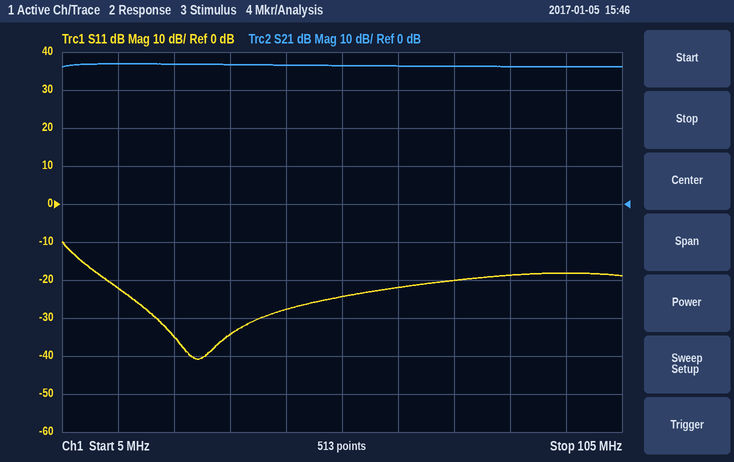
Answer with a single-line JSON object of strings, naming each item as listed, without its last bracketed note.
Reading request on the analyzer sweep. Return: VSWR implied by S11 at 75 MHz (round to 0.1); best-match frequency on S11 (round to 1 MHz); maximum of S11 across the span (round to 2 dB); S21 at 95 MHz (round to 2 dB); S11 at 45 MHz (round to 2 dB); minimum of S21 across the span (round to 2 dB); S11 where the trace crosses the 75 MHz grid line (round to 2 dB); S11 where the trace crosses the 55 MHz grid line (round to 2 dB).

{"VSWR implied by S11 at 75 MHz": "1.2", "best-match frequency on S11": "29 MHz", "maximum of S11 across the span": "-10 dB", "S21 at 95 MHz": "36 dB", "S11 at 45 MHz": "-28 dB", "minimum of S21 across the span": "36 dB", "S11 where the trace crosses the 75 MHz grid line": "-20 dB", "S11 where the trace crosses the 55 MHz grid line": "-24 dB"}
